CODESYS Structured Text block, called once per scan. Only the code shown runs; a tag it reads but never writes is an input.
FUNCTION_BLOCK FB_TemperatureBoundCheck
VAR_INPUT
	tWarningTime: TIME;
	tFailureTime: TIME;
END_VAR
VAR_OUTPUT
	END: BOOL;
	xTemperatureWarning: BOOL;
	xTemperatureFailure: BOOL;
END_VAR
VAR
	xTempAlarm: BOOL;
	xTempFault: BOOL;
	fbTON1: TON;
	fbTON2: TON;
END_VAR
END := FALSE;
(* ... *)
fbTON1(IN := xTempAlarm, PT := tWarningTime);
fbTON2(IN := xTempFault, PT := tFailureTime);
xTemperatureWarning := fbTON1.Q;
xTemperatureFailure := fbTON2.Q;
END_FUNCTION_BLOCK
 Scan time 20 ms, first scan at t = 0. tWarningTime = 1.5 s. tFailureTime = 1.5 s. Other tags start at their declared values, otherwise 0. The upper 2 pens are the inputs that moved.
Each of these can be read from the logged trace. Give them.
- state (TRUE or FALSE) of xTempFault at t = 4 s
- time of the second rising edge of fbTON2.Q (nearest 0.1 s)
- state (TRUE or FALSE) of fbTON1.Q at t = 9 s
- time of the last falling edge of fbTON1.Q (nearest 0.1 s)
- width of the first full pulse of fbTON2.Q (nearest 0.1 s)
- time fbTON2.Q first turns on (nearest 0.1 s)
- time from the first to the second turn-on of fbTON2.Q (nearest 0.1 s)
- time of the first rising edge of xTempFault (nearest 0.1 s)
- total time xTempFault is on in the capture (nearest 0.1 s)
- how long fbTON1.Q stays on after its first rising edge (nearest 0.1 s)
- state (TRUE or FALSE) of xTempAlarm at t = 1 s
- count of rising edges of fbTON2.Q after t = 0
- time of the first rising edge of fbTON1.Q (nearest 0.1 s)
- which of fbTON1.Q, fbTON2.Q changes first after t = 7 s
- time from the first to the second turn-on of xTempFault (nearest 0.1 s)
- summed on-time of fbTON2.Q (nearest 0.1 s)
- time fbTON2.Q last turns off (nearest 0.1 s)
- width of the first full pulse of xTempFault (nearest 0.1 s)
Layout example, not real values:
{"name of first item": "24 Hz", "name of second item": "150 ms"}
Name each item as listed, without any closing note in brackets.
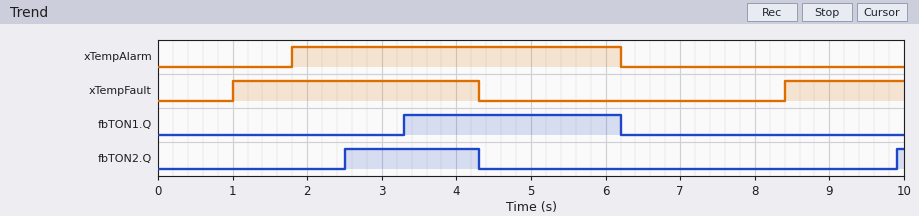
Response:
{"state (TRUE or FALSE) of xTempFault at t = 4 s": "TRUE", "time of the second rising edge of fbTON2.Q": "9.9 s", "state (TRUE or FALSE) of fbTON1.Q at t = 9 s": "FALSE", "time of the last falling edge of fbTON1.Q": "6.2 s", "width of the first full pulse of fbTON2.Q": "1.8 s", "time fbTON2.Q first turns on": "2.5 s", "time from the first to the second turn-on of fbTON2.Q": "7.4 s", "time of the first rising edge of xTempFault": "1.0 s", "total time xTempFault is on in the capture": "4.9 s", "how long fbTON1.Q stays on after its first rising edge": "2.9 s", "state (TRUE or FALSE) of xTempAlarm at t = 1 s": "FALSE", "count of rising edges of fbTON2.Q after t = 0": "2", "time of the first rising edge of fbTON1.Q": "3.3 s", "which of fbTON1.Q, fbTON2.Q changes first after t = 7 s": "fbTON2.Q", "time from the first to the second turn-on of xTempFault": "7.4 s", "summed on-time of fbTON2.Q": "1.9 s", "time fbTON2.Q last turns off": "4.3 s", "width of the first full pulse of xTempFault": "3.3 s"}
